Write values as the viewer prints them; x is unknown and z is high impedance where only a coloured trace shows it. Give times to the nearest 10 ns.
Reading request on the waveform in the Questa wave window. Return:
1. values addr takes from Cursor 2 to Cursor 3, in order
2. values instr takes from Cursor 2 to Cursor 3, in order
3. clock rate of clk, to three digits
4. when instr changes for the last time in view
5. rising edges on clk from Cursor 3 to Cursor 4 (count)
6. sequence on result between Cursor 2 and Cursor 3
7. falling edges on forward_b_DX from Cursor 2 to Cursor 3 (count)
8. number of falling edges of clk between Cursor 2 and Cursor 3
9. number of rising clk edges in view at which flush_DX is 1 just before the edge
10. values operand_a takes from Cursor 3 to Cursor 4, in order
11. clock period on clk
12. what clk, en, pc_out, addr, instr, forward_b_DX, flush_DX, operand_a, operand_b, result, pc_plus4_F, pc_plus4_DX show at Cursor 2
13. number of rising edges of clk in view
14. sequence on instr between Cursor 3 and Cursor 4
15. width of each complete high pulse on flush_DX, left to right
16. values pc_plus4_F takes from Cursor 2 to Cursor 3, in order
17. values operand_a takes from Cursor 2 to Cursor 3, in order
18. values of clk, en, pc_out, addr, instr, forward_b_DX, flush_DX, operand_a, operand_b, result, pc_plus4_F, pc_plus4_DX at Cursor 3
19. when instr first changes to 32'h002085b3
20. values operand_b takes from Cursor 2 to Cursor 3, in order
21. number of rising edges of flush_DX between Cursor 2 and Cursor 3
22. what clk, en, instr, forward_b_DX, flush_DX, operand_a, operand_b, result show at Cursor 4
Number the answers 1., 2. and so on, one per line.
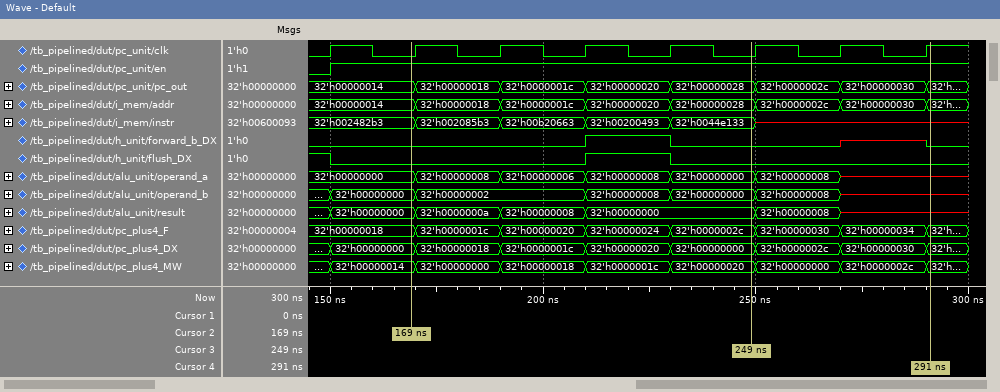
1. 32'h00000014, 32'h00000018, 32'h0000001c, 32'h00000020, 32'h00000028
2. 32'h002482b3, 32'h002085b3, 32'h00b20663, 32'h00200493, 32'h0044e133
3. 50.0 MHz
4. 250 ns
5. 3
6. 32'h00000000, 32'h0000000a, 32'h00000008, 32'h00000000
7. 1
8. 4
9. 2
10. 32'h00000000, 32'h00000008, x
11. 20 ns
12. clk=0, en=1, pc_out=32'h00000014, addr=32'h00000014, instr=32'h002482b3, forward_b_DX=0, flush_DX=0, operand_a=32'h00000000, operand_b=32'h00000000, result=32'h00000000, pc_plus4_F=32'h00000018, pc_plus4_DX=32'h00000000
13. 8
14. 32'h0044e133, x
15. 20 ns
16. 32'h00000018, 32'h0000001c, 32'h00000020, 32'h00000024, 32'h0000002c
17. 32'h00000000, 32'h00000008, 32'h00000006, 32'h00000008, 32'h00000000
18. clk=0, en=1, pc_out=32'h00000028, addr=32'h00000028, instr=32'h0044e133, forward_b_DX=0, flush_DX=0, operand_a=32'h00000000, operand_b=32'h00000000, result=32'h00000000, pc_plus4_F=32'h0000002c, pc_plus4_DX=32'h00000000
19. 170 ns
20. 32'h00000000, 32'h00000002, 32'h00000008, 32'h00000000
21. 1
22. clk=1, en=1, instr=x, forward_b_DX=0, flush_DX=0, operand_a=x, operand_b=x, result=x
